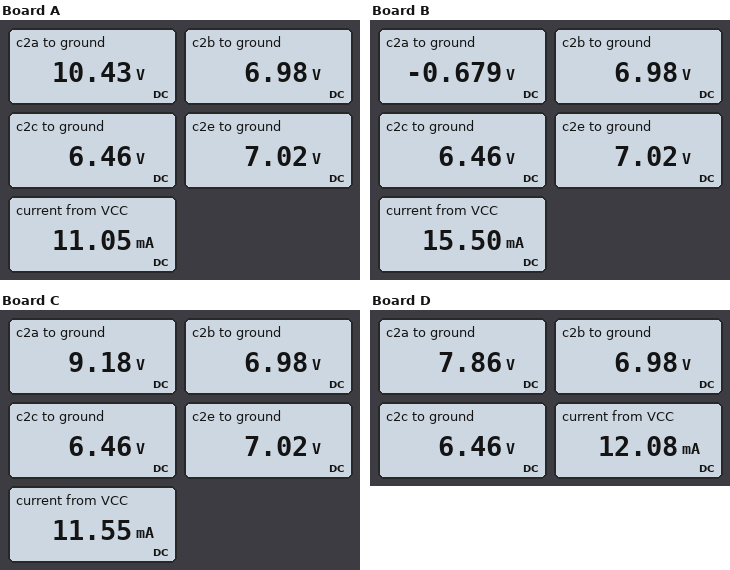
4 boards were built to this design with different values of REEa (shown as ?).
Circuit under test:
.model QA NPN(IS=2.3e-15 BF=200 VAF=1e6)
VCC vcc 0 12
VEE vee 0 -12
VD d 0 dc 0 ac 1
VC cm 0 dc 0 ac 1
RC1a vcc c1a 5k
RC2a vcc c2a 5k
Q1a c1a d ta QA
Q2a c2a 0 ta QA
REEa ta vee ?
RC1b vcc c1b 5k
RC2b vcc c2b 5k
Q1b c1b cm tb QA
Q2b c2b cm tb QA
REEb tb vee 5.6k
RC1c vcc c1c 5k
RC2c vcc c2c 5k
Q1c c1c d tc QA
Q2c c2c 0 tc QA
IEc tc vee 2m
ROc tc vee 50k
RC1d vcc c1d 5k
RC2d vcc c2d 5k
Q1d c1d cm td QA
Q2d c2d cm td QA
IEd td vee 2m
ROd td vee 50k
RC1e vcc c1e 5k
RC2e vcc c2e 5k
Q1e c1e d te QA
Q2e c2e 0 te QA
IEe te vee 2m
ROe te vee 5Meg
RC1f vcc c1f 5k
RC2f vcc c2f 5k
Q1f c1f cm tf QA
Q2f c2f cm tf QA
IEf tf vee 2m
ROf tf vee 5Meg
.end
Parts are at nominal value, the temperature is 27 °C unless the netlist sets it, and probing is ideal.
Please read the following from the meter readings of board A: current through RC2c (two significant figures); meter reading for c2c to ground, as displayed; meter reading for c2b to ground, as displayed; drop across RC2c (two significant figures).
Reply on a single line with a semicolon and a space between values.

1.1 mA; 6.46 V; 6.98 V; 5.5 V
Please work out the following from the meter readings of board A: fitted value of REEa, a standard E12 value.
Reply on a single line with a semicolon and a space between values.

18 kΩ
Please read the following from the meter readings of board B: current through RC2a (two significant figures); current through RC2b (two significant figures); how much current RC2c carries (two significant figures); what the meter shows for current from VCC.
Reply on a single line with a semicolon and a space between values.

2.5 mA; 1.0 mA; 1.1 mA; 15.50 mA
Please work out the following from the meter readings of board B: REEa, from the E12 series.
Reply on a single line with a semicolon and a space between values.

1.8 kΩ
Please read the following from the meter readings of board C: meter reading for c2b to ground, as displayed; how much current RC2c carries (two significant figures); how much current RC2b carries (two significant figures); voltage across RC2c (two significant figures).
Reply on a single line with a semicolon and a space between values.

6.98 V; 1.1 mA; 1.0 mA; 5.5 V
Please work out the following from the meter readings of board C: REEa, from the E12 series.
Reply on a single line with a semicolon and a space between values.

10 kΩ
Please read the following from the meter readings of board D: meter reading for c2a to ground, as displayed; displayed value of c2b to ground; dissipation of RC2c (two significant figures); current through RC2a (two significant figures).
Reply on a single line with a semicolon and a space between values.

7.86 V; 6.98 V; 6.1 mW; 830 µA
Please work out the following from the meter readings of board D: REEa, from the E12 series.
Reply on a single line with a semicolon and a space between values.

6.8 kΩ
